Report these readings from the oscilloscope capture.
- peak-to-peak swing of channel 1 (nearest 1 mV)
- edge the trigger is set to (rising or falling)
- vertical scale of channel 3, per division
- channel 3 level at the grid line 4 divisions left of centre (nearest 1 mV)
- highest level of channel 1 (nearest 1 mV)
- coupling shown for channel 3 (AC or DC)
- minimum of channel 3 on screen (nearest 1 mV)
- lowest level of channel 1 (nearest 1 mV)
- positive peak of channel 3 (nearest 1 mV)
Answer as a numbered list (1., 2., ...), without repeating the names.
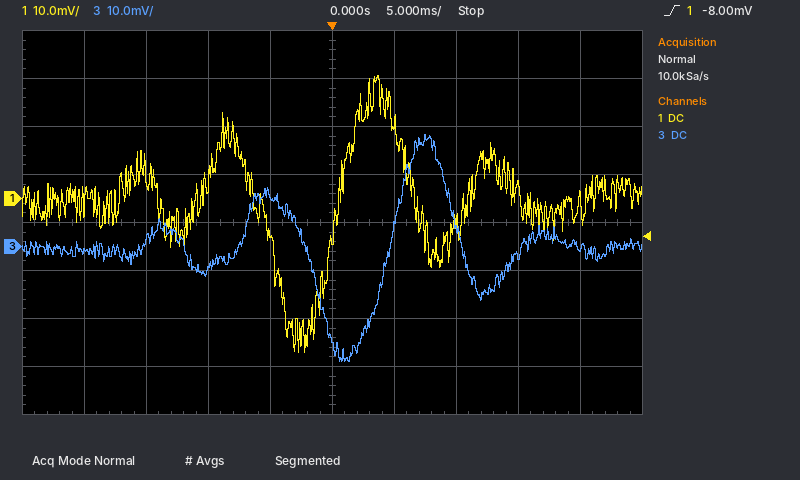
1. 58 mV
2. rising
3. 10 mV
4. -1 mV
5. 26 mV
6. DC
7. -24 mV
8. -32 mV
9. 23 mV
